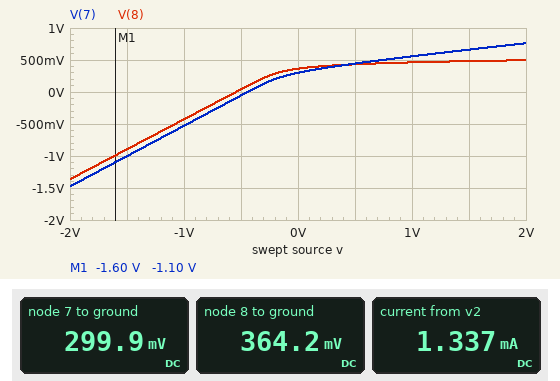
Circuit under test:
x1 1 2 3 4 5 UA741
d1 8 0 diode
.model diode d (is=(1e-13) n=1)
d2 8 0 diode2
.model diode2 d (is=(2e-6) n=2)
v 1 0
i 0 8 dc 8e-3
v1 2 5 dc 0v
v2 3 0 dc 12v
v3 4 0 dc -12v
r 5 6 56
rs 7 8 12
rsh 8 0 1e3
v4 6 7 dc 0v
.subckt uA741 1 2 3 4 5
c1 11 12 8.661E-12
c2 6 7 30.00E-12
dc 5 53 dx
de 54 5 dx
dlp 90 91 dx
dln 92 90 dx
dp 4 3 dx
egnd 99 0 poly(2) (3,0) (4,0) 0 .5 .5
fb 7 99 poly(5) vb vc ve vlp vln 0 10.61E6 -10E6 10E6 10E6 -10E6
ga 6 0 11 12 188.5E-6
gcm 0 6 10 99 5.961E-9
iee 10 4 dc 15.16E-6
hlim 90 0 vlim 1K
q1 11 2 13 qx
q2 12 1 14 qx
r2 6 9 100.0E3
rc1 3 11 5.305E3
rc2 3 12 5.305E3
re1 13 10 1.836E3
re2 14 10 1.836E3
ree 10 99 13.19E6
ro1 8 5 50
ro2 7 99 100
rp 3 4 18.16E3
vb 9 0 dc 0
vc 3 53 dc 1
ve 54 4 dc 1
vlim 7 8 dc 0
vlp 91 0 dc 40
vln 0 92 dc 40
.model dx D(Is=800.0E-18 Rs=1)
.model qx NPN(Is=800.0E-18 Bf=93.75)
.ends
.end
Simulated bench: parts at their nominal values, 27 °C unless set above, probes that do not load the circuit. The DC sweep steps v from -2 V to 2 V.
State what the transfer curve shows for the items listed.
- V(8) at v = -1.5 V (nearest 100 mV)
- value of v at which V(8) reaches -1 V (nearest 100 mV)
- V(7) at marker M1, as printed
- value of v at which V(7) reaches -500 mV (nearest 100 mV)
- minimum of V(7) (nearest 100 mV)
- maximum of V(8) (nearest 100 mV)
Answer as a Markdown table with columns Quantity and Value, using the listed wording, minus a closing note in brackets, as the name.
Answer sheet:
| Quantity | Value |
|---|---|
| V(8) at v = -1.5 V | -900 mV |
| value of v at which V(8) reaches -1 V | -1.6 V |
| V(7) at marker M1, as printed | -1.10 V |
| value of v at which V(7) reaches -500 mV | -1.0 V |
| minimum of V(7) | -1.5 V |
| maximum of V(8) | 500 mV |
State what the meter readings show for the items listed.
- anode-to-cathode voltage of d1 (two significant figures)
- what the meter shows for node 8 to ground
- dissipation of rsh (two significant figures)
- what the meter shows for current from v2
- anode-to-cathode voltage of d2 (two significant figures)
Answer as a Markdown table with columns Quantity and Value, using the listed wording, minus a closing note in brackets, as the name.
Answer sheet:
| Quantity | Value |
|---|---|
| anode-to-cathode voltage of d1 | 360 mV |
| what the meter shows for node 8 to ground | 364.2 mV |
| dissipation of rsh | 130 µW |
| what the meter shows for current from v2 | 1.337 mA |
| anode-to-cathode voltage of d2 | 360 mV |
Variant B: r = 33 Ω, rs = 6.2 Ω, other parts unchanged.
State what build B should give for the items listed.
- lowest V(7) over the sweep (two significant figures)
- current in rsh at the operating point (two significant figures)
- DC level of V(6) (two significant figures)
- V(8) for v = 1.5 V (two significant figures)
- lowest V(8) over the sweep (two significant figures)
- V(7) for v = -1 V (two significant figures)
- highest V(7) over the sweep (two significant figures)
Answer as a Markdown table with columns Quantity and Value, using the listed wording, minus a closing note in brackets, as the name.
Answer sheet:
| Quantity | Value |
|---|---|
| lowest V(7) over the sweep | -1.7 V |
| current in rsh at the operating point | 280 µA |
| DC level of V(6) | 240 mV |
| V(8) for v = 1.5 V | 500 mV |
| lowest V(8) over the sweep | -1.6 V |
| V(7) for v = -1 V | -710 mV |
| highest V(7) over the sweep | 750 mV |
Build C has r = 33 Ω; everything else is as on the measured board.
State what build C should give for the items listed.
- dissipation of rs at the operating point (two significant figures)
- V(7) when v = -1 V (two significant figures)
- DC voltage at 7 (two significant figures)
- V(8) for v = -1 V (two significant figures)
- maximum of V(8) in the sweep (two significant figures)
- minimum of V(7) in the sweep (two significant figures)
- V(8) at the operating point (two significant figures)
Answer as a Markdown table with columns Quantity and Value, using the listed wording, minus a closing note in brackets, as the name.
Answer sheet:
| Quantity | Value |
|---|---|
| dissipation of rs at the operating point | 570 µW |
| V(7) when v = -1 V | -720 mV |
| DC voltage at 7 | 230 mV |
| V(8) for v = -1 V | -610 mV |
| maximum of V(8) in the sweep | 510 mV |
| minimum of V(7) in the sweep | -1.7 V |
| V(8) at the operating point | 310 mV |
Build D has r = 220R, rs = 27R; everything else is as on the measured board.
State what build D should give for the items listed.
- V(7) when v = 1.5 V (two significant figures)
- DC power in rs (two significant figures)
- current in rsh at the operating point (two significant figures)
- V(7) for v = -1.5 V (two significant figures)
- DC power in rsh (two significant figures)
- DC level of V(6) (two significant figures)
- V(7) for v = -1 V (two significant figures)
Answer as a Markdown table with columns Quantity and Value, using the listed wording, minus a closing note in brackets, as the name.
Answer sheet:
| Quantity | Value |
|---|---|
| V(7) when v = 1.5 V | 560 mV |
| DC power in rs | 76 µW |
| current in rsh at the operating point | 410 µA |
| V(7) for v = -1.5 V | 90 mV |
| DC power in rsh | 170 µW |
| DC level of V(6) | 370 mV |
| V(7) for v = -1 V | 210 mV |
